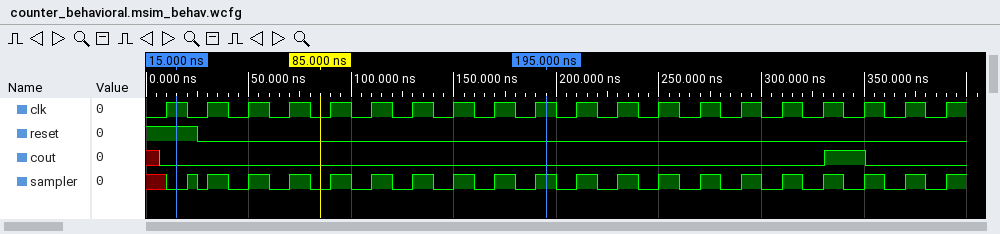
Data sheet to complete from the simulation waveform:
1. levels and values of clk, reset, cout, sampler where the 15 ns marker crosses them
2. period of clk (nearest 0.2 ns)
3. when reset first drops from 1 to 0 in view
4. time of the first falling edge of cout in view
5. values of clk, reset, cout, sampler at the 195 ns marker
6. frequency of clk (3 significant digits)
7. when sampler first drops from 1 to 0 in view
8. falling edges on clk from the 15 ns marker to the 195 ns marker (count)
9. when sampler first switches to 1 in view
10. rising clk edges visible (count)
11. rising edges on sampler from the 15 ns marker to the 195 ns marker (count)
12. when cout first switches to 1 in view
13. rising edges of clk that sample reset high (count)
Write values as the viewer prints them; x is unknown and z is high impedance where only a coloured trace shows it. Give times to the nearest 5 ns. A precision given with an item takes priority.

clk=1, reset=1, cout=0, sampler=0
20 ns
25 ns
350 ns
clk=1, reset=0, cout=0, sampler=1
50.0 MHz
25 ns
9
20 ns
20
10
330 ns
1
